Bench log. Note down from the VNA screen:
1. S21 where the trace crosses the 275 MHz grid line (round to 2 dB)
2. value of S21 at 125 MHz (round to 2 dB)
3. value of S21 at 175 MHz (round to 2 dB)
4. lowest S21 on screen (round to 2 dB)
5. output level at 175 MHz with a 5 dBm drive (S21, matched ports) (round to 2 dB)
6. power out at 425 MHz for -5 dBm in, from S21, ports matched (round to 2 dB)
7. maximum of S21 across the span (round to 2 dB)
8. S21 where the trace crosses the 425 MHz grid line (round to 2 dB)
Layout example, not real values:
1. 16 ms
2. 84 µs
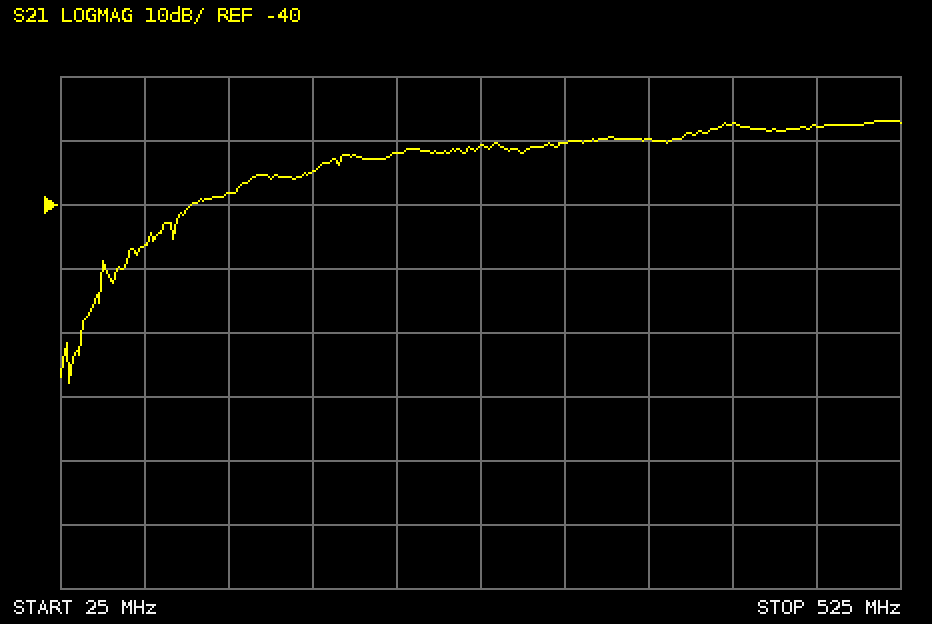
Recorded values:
1. -30 dB
2. -38 dB
3. -34 dB
4. -68 dB
5. -30 dBm
6. -32 dBm
7. -26 dB
8. -28 dB
